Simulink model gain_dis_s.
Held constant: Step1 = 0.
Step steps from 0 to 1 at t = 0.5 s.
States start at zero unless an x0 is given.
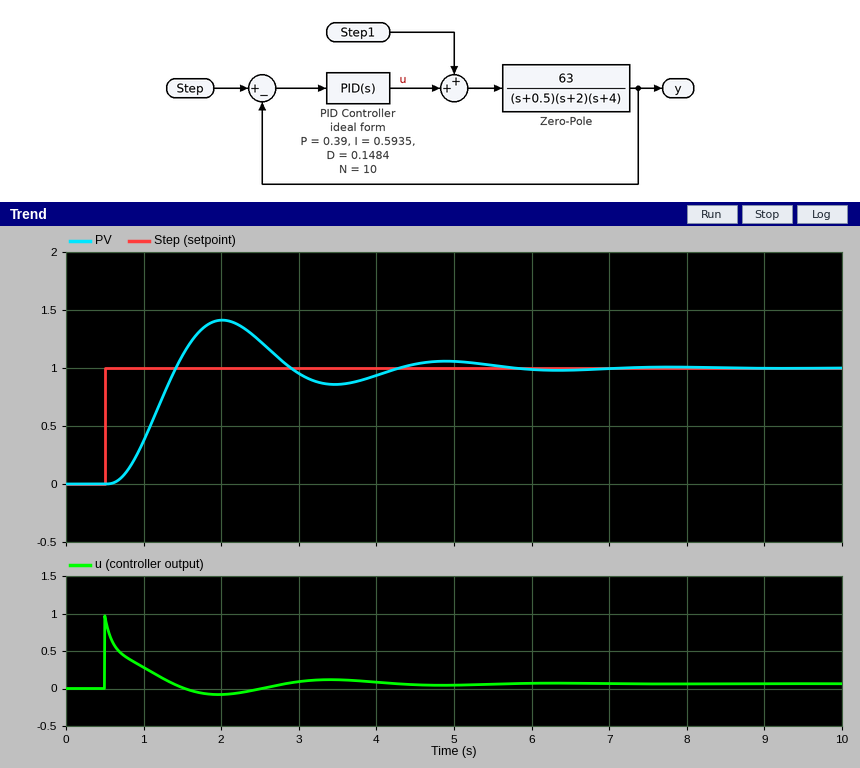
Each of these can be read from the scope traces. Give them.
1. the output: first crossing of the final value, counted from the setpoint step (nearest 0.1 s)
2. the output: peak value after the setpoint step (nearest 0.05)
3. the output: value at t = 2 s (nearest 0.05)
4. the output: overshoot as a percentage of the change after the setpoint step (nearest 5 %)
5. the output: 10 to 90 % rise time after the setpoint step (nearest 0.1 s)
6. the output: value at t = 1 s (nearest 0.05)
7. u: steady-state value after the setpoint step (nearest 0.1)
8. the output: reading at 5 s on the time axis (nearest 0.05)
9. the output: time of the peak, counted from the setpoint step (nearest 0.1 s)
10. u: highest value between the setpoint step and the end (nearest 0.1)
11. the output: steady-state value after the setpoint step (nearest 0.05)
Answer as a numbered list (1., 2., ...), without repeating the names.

1. 0.9 s
2. 1.40
3. 1.40
4. 40 %
5. 0.6 s
6. 0.35
7. 0.1
8. 1.05
9. 1.5 s
10. 1.0
11. 1.00
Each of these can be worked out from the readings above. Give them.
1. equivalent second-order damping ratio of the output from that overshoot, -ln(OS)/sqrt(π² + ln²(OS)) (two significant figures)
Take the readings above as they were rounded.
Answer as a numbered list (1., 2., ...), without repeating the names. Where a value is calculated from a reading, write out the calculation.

1. ln(0.4) = -0.916; 0.916 / sqrt(9.870 + 0.840) = 0.28
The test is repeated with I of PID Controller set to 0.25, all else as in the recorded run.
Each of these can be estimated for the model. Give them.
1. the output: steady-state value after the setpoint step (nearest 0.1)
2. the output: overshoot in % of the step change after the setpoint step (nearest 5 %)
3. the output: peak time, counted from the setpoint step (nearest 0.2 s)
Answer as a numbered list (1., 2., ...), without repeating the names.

1. 1.0
2. 25 %
3. 1.4 s
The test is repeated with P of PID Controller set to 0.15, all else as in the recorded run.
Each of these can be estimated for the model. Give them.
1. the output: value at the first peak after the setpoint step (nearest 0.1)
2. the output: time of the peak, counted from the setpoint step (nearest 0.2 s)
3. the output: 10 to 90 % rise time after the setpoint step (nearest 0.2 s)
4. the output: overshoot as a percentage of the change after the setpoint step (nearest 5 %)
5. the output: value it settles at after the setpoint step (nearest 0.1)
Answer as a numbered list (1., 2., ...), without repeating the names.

1. 1.2
2. 2.8 s
3. 1.2 s
4. 15 %
5. 1.0
